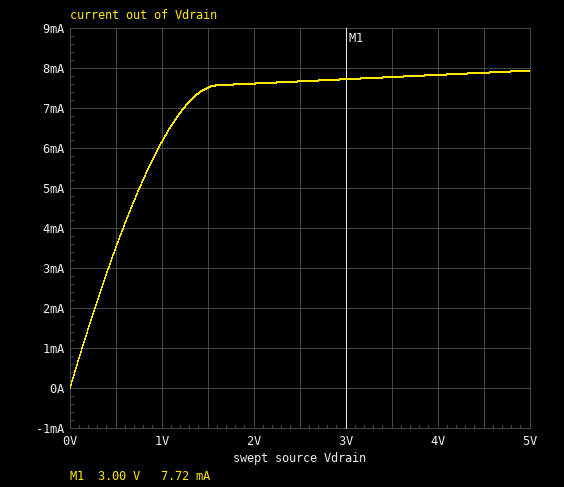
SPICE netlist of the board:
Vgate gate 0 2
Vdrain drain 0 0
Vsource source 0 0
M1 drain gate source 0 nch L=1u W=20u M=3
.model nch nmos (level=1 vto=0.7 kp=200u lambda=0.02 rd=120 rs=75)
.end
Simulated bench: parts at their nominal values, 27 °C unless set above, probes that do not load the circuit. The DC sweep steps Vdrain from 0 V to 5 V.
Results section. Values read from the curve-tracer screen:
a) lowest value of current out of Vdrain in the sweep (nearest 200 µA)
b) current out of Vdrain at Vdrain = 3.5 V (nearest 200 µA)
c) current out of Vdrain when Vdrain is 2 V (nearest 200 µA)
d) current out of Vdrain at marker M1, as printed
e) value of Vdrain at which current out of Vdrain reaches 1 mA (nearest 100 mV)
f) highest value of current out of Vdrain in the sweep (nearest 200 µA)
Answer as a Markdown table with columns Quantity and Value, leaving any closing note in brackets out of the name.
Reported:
| Quantity | Value |
|---|---|
| lowest value of current out of Vdrain in the sweep | 0 A |
| current out of Vdrain at Vdrain = 3.5 V | 7.8 mA |
| current out of Vdrain when Vdrain is 2 V | 7.6 mA |
| current out of Vdrain at marker M1, as printed | 7.72 mA |
| value of Vdrain at which current out of Vdrain reaches 1 mA | 100 mV |
| highest value of current out of Vdrain in the sweep | 8.0 mA |
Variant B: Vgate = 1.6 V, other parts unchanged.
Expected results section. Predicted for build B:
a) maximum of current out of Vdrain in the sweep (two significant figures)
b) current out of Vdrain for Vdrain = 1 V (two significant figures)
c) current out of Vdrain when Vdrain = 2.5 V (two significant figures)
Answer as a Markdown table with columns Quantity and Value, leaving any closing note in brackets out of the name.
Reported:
| Quantity | Value |
|---|---|
| maximum of current out of Vdrain in the sweep | 4.2 mA |
| current out of Vdrain for Vdrain = 1 V | 3.9 mA |
| current out of Vdrain when Vdrain = 2.5 V | 4.0 mA |
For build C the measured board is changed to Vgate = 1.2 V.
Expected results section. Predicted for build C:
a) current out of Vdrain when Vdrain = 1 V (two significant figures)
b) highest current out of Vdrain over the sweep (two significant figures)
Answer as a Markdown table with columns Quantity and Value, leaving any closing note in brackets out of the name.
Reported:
| Quantity | Value |
|---|---|
| current out of Vdrain when Vdrain = 1 V | 1.3 mA |
| highest current out of Vdrain over the sweep | 1.4 mA |
